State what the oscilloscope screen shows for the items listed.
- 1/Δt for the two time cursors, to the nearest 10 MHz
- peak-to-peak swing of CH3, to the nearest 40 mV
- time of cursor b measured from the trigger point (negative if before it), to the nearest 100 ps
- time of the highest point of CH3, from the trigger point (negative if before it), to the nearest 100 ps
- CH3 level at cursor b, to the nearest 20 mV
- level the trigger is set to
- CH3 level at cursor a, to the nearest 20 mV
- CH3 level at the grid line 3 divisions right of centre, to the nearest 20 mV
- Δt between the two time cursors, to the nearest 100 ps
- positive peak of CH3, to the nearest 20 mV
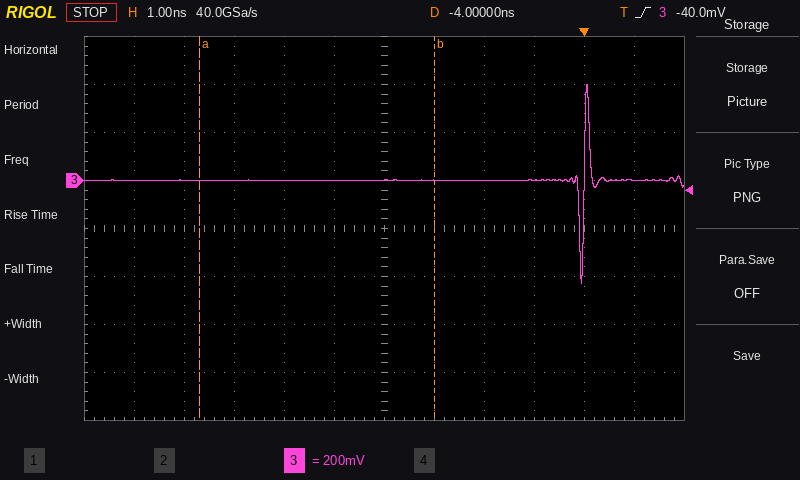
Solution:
210 MHz
840 mV
-3.0 ns
+100 ps
0 mV
-40.0 mV
0 mV
0 mV
4.7 ns
400 mV
